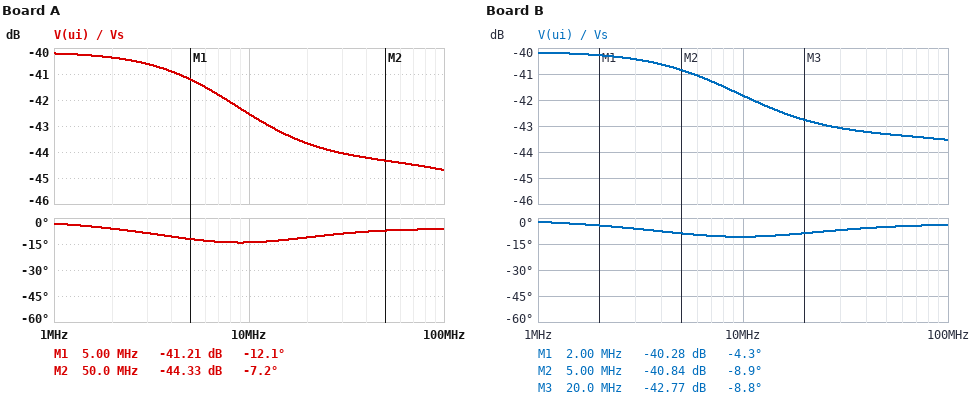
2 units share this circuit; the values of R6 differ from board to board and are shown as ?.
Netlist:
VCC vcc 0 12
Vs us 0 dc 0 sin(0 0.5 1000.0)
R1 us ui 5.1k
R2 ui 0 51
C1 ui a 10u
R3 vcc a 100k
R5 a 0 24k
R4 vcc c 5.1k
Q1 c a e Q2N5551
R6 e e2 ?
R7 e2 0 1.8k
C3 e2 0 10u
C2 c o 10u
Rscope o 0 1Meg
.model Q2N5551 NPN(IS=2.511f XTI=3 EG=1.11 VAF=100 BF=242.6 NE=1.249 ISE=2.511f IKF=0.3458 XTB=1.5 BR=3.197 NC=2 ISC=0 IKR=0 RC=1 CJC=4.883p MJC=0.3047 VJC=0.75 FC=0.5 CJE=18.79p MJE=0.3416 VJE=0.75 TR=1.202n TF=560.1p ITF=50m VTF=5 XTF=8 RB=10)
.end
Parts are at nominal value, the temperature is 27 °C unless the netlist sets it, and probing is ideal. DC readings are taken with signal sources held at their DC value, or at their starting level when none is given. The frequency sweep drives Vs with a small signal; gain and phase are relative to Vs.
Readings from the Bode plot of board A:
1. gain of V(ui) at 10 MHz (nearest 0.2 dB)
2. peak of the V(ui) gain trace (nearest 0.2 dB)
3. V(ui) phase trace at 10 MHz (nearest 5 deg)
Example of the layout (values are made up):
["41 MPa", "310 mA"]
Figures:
["-42.6 dB", "-40.2 dB", "-15 deg"]
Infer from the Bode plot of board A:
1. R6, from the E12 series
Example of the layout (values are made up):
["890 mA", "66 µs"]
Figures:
["47 Ω"]
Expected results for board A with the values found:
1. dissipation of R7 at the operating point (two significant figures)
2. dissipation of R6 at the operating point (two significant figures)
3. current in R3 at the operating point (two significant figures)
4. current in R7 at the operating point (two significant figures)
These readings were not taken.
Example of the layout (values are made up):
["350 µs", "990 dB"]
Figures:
["1.2 mW", "31 µW", "98 µA", "810 µA"]
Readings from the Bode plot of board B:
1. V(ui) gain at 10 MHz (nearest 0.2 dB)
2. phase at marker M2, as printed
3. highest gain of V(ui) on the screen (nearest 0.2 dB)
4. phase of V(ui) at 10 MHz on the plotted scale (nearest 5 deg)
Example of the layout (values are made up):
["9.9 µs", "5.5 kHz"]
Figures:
["-41.8 dB", "-8.9 deg", "-40.2 dB", "-10 deg"]
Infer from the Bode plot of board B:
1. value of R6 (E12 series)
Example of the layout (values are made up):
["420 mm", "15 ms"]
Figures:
["82 Ω"]
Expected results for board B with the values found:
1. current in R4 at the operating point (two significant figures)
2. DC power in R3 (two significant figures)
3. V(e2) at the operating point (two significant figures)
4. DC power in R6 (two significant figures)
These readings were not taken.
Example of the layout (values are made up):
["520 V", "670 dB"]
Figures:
["790 µA", "960 µW", "1.4 V", "52 µW"]
